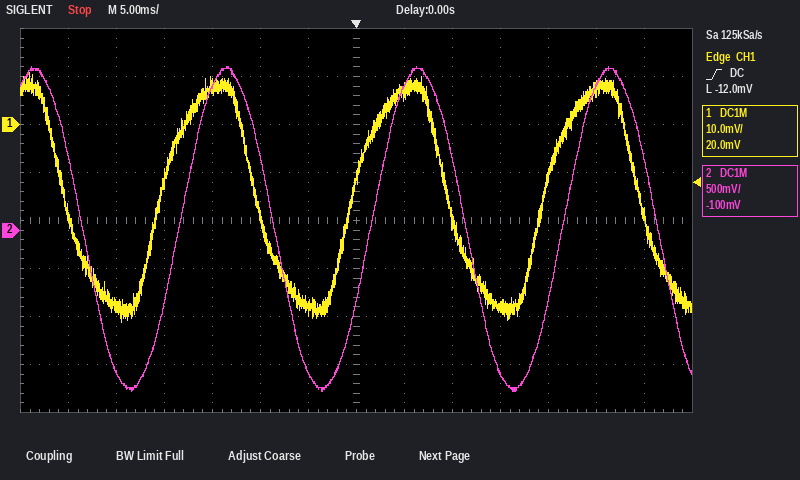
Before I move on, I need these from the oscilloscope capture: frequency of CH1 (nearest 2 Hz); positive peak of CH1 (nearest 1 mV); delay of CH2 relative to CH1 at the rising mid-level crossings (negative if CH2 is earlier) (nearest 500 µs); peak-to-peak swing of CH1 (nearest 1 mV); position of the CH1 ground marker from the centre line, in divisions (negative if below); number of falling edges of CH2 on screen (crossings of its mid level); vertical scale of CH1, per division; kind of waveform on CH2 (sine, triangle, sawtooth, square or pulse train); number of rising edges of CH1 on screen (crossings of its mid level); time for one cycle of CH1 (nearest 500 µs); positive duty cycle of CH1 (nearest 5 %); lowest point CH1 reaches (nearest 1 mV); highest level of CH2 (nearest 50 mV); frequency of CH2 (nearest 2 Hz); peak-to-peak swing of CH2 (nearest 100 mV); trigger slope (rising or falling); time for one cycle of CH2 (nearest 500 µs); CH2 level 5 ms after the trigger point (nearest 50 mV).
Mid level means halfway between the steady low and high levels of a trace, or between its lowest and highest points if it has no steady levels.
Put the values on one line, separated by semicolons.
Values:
50 Hz; 11 mV; +2.0 ms; 52 mV; +2.0 div; 4; 10 mV; sine; 3; 20.0 ms; 50 %; -41 mV; 1.70 V; 50 Hz; 3.40 V; rising; 20.0 ms; 1.50 V
